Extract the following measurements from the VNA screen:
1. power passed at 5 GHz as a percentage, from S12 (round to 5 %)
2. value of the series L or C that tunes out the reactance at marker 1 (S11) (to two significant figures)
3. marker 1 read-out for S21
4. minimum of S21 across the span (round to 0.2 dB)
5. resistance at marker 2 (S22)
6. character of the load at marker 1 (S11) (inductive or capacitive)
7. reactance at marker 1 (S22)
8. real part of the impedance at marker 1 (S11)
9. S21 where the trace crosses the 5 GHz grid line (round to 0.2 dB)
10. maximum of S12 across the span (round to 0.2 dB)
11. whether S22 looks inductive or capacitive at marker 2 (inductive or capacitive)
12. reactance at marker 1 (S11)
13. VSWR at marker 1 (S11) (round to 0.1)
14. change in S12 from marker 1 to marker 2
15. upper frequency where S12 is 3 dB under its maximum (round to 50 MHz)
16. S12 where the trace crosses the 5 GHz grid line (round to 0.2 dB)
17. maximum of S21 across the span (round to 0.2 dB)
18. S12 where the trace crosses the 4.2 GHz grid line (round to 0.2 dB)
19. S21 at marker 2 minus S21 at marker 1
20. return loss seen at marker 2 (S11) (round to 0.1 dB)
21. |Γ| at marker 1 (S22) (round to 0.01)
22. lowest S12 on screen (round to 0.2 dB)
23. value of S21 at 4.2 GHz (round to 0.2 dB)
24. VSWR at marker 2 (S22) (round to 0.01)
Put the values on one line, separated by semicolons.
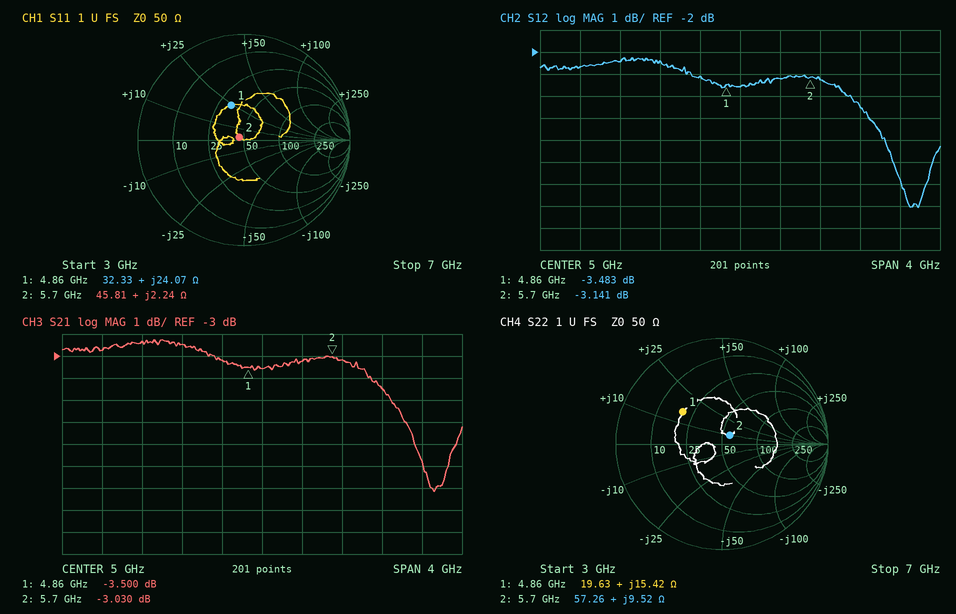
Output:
45 %; 1.4 pF; -3.500 dB; -9.2 dB; 57.26 Ω; inductive; +15.42 Ω; 32.33 Ω; -3.6 dB; -2.2 dB; inductive; +24.07 Ω; 2.1; 0.342 dB; 6.35 GHz; -3.6 dB; -2.2 dB; -2.4 dB; 0.470 dB; 26.1 dB; 0.48; -9.0 dB; -2.4 dB; 1.25
